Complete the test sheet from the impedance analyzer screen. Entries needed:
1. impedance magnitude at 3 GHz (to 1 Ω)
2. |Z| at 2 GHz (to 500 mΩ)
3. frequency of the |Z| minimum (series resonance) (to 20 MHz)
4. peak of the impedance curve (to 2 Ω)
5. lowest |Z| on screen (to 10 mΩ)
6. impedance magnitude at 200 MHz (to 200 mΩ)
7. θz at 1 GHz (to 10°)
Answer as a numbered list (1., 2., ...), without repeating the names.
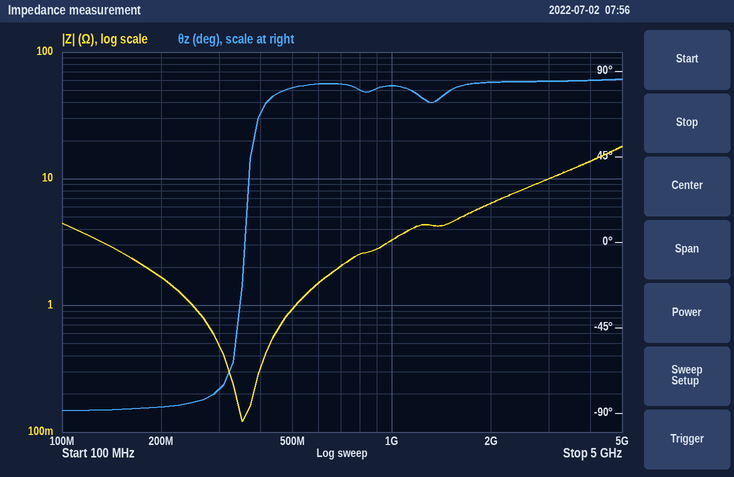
1. 10 Ω
2. 6.5 Ω
3. 360 MHz
4. 18 Ω
5. 120 mΩ
6. 1.6 Ω
7. 80°
